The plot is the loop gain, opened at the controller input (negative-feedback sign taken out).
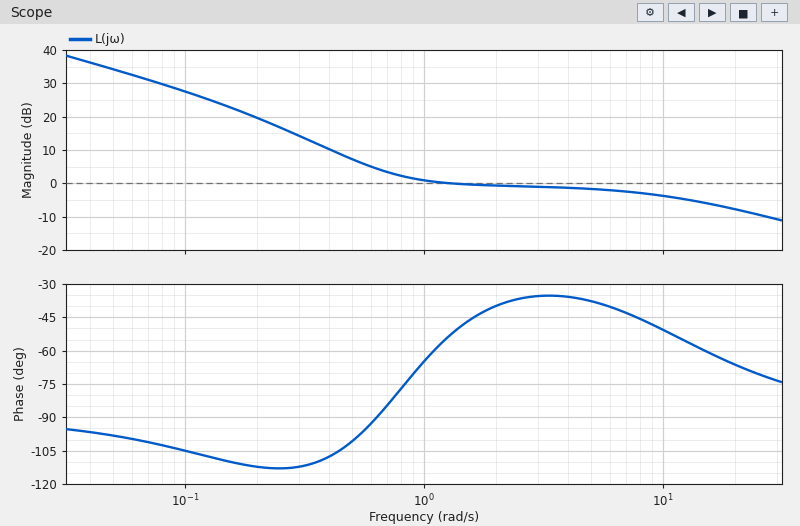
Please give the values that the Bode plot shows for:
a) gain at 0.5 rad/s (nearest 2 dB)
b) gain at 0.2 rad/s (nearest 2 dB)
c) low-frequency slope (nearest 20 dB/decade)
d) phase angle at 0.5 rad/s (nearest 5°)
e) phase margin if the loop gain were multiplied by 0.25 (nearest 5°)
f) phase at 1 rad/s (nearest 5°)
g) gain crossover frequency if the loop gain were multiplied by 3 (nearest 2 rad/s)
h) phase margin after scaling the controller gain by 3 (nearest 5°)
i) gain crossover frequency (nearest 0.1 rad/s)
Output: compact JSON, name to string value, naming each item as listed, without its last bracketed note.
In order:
{"gain at 0.5 rad/s": "8 dB", "gain at 0.2 rad/s": "20 dB", "low-frequency slope": "-20 dB/decade", "phase angle at 0.5 rad/s": "-100°", "phase margin if the loop gain were multiplied by 0.25": "70°", "phase at 1 rad/s": "-65°", "gain crossover frequency if the loop gain were multiplied by 3": "26 rad/s", "phase margin after scaling the controller gain by 3": "110°", "gain crossover frequency": "1.3 rad/s"}
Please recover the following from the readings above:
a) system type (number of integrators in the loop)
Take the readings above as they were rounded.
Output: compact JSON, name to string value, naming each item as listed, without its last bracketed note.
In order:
{"system type": "1"}
